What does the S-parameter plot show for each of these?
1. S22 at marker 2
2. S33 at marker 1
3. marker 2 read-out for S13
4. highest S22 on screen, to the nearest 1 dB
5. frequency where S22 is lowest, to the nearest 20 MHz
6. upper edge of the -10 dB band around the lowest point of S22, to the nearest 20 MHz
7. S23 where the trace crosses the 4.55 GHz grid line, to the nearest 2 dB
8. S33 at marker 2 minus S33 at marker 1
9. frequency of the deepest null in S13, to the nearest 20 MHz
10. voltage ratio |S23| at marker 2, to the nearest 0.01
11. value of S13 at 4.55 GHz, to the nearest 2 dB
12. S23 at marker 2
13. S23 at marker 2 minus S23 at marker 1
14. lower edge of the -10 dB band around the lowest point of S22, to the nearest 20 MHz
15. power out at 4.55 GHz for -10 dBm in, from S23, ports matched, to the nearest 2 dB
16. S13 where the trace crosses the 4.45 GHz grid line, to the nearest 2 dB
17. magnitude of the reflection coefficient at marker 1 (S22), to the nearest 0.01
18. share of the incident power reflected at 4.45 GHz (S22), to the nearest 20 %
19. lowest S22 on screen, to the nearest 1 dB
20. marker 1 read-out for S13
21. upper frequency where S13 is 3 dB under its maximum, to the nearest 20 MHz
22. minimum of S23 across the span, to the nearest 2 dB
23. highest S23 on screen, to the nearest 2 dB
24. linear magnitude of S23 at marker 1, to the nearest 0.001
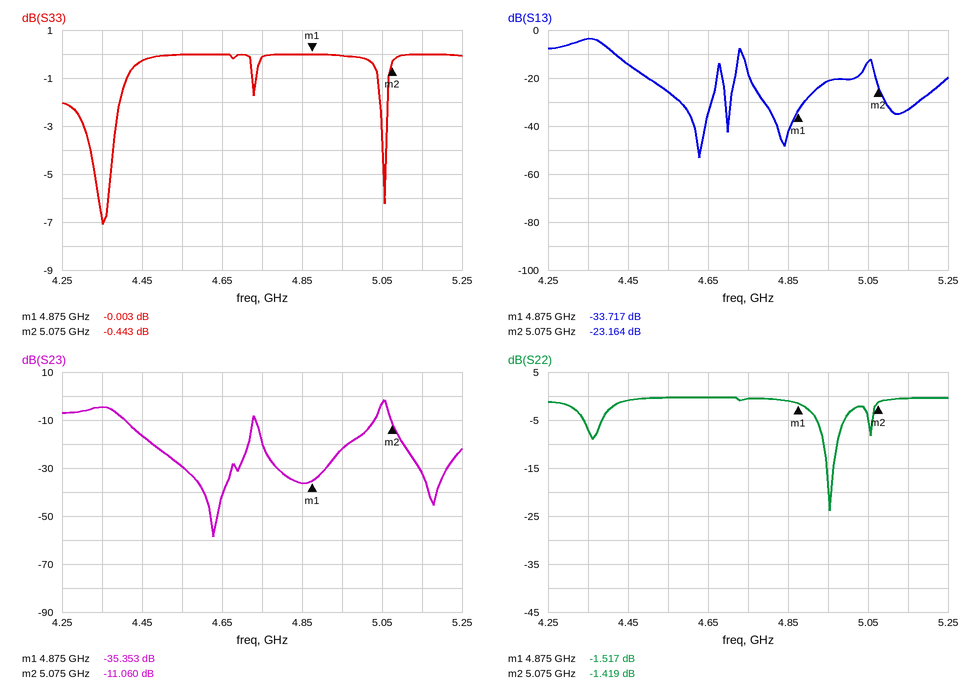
-1.419 dB
-0.003 dB
-23.164 dB
0 dB
4.96 GHz
4.98 GHz
-30 dB
-0.440 dB
4.62 GHz
0.28
-26 dB
-11.060 dB
24.293 dB
4.94 GHz
-40 dBm
-14 dB
0.84
80 %
-24 dB
-33.717 dB
4.40 GHz
-58 dB
-2 dB
0.017
